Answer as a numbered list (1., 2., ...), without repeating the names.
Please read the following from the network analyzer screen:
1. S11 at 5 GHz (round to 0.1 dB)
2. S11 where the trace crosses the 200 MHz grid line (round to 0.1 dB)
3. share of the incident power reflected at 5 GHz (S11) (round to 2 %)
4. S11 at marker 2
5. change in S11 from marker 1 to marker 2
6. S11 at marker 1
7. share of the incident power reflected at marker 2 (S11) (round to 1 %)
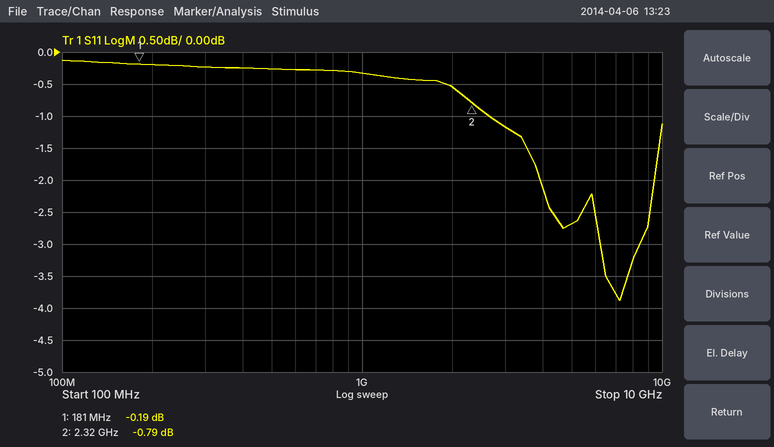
1. -2.7 dB
2. -0.2 dB
3. 54 %
4. -0.79 dB
5. -0.60 dB
6. -0.19 dB
7. 83 %
